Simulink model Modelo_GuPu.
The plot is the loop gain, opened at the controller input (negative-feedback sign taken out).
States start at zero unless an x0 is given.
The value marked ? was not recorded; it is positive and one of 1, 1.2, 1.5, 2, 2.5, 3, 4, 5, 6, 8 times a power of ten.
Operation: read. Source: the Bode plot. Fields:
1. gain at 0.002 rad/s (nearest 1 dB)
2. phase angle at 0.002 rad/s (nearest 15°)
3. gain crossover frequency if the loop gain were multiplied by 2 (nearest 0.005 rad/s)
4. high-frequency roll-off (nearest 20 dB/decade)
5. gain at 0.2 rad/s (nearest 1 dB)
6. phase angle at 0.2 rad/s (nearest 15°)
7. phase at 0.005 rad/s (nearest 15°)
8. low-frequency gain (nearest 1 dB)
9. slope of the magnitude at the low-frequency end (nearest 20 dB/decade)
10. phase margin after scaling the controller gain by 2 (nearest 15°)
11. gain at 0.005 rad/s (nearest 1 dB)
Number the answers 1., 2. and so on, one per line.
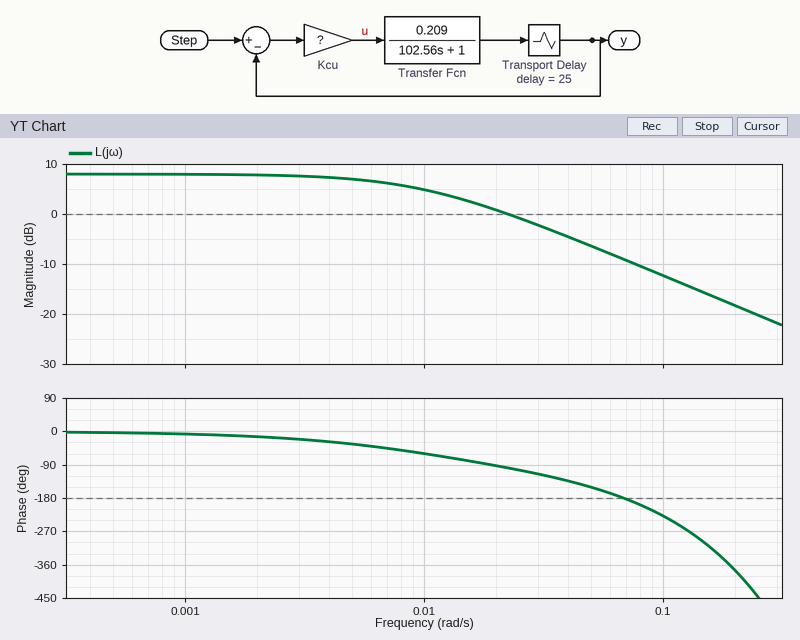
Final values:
1. 8 dB
2. -15°
3. 0.050 rad/s
4. -20 dB/decade
5. -18 dB
6. -375°
7. -30°
8. 8 dB
9. 0 dB/decade
10. 30°
11. 7 dB
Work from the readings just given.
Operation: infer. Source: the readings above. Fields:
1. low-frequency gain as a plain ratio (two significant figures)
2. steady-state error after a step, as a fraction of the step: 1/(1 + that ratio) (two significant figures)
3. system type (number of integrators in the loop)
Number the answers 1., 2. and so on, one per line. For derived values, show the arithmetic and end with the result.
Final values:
1. 10^(8 / 20) = 2.5
2. 1 / (1 + 2.5) = 0.29
3. 0
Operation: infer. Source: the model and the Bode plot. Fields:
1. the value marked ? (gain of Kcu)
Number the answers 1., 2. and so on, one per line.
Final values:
1. 12
